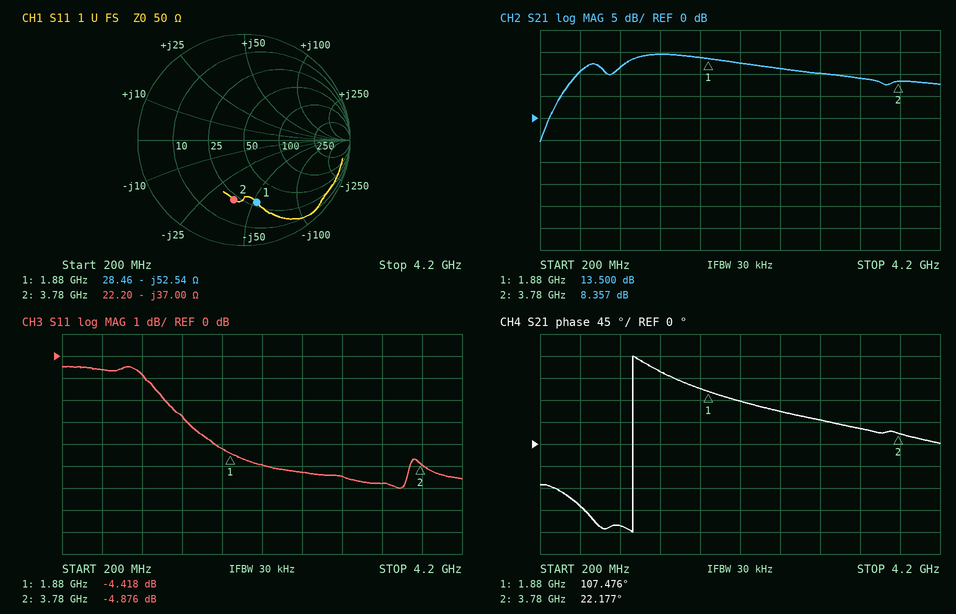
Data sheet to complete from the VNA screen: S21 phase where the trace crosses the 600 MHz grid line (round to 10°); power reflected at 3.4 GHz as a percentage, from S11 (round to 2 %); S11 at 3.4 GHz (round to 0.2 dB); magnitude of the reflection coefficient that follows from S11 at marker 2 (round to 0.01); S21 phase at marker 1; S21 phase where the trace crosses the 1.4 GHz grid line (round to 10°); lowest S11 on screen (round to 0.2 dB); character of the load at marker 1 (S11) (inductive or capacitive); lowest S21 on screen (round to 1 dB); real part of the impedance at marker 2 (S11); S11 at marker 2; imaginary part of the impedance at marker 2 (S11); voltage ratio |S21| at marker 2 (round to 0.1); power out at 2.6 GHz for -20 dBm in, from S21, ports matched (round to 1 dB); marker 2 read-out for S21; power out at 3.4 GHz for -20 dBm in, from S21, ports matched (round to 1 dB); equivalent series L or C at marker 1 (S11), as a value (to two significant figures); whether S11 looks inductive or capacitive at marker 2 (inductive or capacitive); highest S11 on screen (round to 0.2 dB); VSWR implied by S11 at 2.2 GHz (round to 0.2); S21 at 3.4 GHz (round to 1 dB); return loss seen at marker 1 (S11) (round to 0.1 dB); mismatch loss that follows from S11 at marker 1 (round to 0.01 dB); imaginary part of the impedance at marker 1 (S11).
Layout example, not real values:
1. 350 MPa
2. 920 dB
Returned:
1. -130°
2. 26 %
3. -5.8 dB
4. 0.57
5. 107.476°
6. 150°
7. -6.0 dB
8. capacitive
9. -5 dB
10. 22.20 Ω
11. -4.876 dB
12. -37.00 Ω
13. 2.6
14. -9 dBm
15. 8.357 dB
16. -11 dBm
17. 1.6 pF
18. capacitive
19. -0.4 dB
20. 3.6
21. 9 dB
22. 4.4 dB
23. 1.95 dB
24. -52.54 Ω
